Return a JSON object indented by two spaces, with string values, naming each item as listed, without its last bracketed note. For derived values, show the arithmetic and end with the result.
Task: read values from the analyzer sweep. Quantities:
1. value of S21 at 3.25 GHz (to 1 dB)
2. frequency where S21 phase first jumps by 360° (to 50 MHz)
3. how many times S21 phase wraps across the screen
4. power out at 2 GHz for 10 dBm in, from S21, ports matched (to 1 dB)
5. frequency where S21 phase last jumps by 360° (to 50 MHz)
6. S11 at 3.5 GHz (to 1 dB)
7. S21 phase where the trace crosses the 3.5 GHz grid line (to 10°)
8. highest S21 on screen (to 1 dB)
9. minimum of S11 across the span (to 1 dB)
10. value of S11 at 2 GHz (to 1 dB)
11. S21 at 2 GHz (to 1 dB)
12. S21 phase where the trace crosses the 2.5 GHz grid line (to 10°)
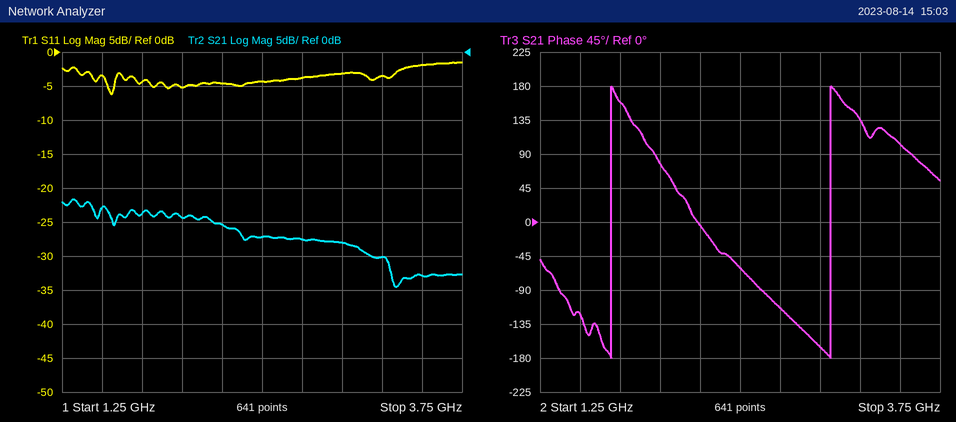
{
  "value of S21 at 3.25 GHz": "-30 dB",
  "frequency where S21 phase first jumps by 360°": "1.70 GHz",
  "how many times S21 phase wraps across the screen": "2",
  "power out at 2 GHz for 10 dBm in, from S21, ports matched": "10 dBm + (-24 dB) = -14 dBm",
  "frequency where S21 phase last jumps by 360°": "3.05 GHz",
  "S11 at 3.5 GHz": "-2 dB",
  "S21 phase where the trace crosses the 3.5 GHz grid line": "100°",
  "highest S21 on screen": "-22 dB",
  "minimum of S11 across the span": "-6 dB",
  "value of S11 at 2 GHz": "-5 dB",
  "S21 at 2 GHz": "-24 dB",
  "S21 phase where the trace crosses the 2.5 GHz grid line": "-60°"
}
